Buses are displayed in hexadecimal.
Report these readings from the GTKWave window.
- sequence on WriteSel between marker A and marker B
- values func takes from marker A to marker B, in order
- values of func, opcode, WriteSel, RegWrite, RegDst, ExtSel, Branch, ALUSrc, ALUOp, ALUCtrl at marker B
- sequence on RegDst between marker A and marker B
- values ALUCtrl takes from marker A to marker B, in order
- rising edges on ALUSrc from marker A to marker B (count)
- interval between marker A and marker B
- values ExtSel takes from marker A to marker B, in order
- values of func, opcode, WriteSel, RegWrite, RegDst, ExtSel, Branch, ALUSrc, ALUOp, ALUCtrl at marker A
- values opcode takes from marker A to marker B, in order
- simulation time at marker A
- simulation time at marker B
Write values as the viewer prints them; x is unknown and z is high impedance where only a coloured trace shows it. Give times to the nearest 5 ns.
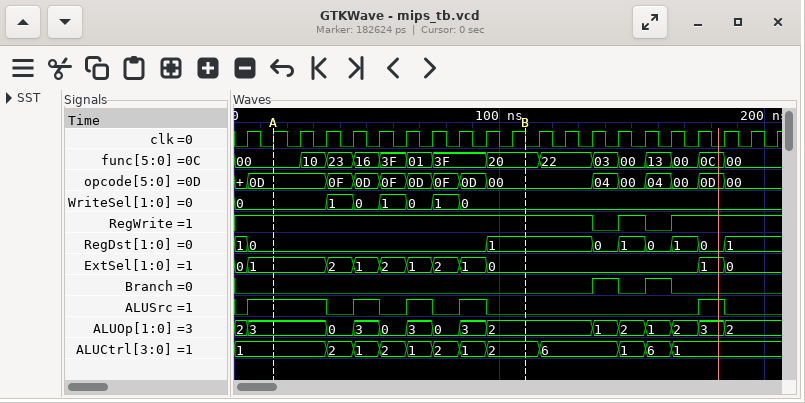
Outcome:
0, 1, 0, 1, 0, 1, 0
00, 10, 23, 16, 3F, 01, 3F, 20
func=20, opcode=00, WriteSel=0, RegWrite=1, RegDst=1, ExtSel=0, Branch=0, ALUSrc=0, ALUOp=2, ALUCtrl=2
0, 1
1, 2, 1, 2, 1, 2, 1, 2
3
95 ns
1, 2, 1, 2, 1, 2, 1, 0
func=00, opcode=0D, WriteSel=0, RegWrite=1, RegDst=0, ExtSel=1, Branch=0, ALUSrc=1, ALUOp=3, ALUCtrl=1
0D, 0F, 0D, 0F, 0D, 0F, 0D, 00
15 ns
110 ns
